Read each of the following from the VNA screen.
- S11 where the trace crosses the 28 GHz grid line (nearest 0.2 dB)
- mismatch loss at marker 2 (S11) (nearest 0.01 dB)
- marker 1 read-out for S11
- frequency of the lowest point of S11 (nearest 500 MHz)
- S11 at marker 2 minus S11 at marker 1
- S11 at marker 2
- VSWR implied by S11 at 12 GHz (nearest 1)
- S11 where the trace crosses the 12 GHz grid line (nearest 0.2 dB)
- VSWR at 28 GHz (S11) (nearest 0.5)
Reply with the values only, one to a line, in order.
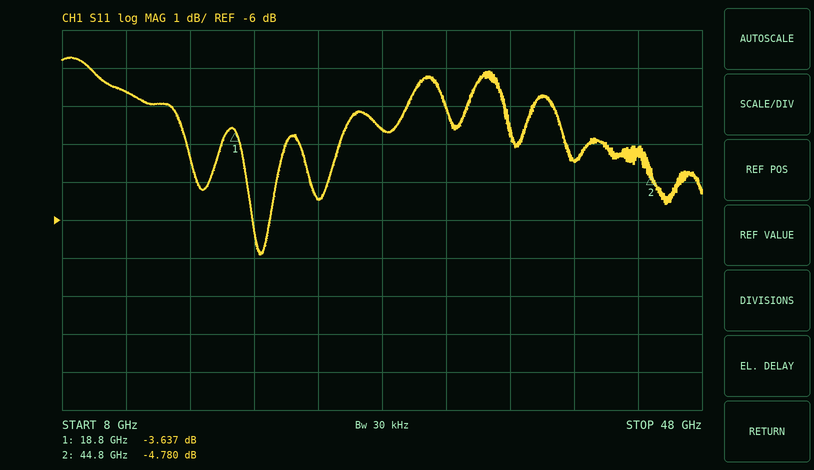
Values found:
-3.6 dB
1.76 dB
-3.637 dB
20.5 GHz
-1.143 dB
-4.780 dB
7
-2.6 dB
5.0
